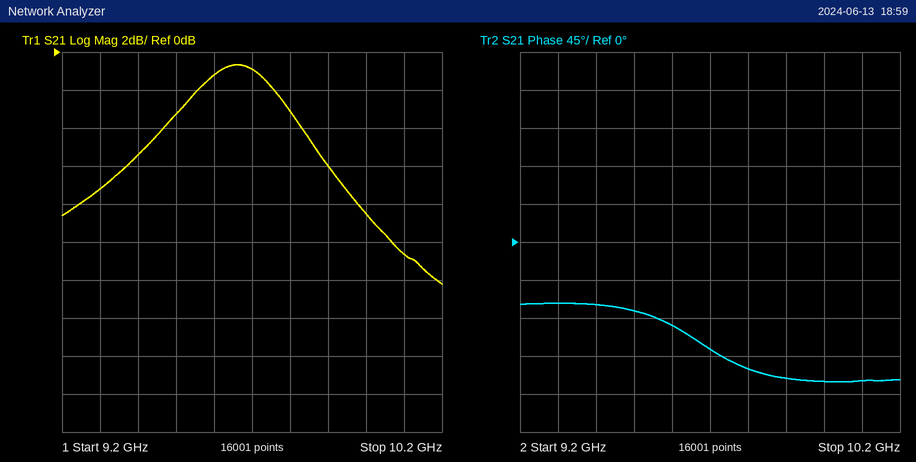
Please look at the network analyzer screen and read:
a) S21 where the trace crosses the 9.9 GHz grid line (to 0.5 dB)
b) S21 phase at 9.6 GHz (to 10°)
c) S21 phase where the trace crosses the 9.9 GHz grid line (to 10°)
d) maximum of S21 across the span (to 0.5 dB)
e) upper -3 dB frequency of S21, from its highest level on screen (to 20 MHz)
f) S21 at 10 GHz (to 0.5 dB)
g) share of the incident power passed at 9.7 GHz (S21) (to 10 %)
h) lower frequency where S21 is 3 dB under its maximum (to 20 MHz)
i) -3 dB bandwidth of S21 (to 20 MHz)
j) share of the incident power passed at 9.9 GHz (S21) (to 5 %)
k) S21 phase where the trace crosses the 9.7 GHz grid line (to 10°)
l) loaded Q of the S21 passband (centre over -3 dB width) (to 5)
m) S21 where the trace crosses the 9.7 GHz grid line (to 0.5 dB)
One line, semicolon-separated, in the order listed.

-6.0 dB; -100°; -160°; -0.5 dB; 9.82 GHz; -8.5 dB; 80 %; 9.48 GHz; 340 MHz; 25 %; -130°; 30; -1.0 dB
